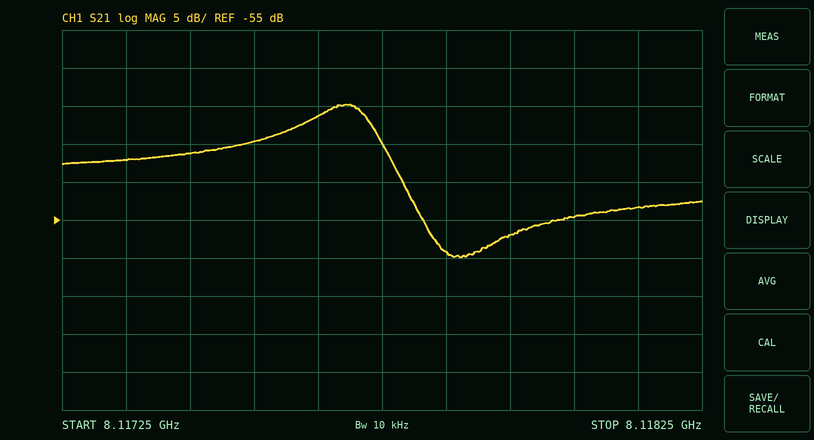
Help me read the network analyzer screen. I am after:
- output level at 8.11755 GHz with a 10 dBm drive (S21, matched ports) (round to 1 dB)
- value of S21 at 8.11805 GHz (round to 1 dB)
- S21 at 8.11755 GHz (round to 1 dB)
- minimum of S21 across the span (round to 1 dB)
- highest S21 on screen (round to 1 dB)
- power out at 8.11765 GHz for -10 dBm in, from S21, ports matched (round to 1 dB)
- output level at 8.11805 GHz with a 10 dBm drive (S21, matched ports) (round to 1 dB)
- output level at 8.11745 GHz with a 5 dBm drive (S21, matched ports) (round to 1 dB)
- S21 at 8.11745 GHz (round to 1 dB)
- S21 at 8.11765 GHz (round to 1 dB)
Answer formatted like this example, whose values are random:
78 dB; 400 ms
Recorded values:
-35 dBm; -55 dB; -45 dB; -60 dB; -40 dB; -51 dBm; -45 dBm; -41 dBm; -46 dB; -41 dB
